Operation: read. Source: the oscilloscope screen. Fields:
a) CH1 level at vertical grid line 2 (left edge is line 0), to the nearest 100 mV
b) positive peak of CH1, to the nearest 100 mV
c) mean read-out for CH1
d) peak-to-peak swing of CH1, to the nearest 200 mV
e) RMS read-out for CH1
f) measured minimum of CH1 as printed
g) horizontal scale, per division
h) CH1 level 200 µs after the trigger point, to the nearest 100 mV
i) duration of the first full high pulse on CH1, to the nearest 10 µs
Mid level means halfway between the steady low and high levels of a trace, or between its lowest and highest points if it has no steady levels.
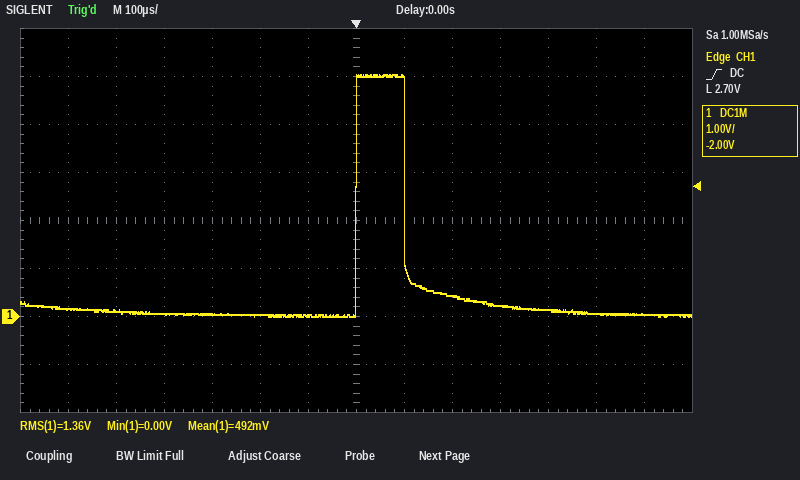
100 mV
5.0 V
492 mV
5.0 V
1.36 V
0.00 V
100 µs
400 mV
100 µs
